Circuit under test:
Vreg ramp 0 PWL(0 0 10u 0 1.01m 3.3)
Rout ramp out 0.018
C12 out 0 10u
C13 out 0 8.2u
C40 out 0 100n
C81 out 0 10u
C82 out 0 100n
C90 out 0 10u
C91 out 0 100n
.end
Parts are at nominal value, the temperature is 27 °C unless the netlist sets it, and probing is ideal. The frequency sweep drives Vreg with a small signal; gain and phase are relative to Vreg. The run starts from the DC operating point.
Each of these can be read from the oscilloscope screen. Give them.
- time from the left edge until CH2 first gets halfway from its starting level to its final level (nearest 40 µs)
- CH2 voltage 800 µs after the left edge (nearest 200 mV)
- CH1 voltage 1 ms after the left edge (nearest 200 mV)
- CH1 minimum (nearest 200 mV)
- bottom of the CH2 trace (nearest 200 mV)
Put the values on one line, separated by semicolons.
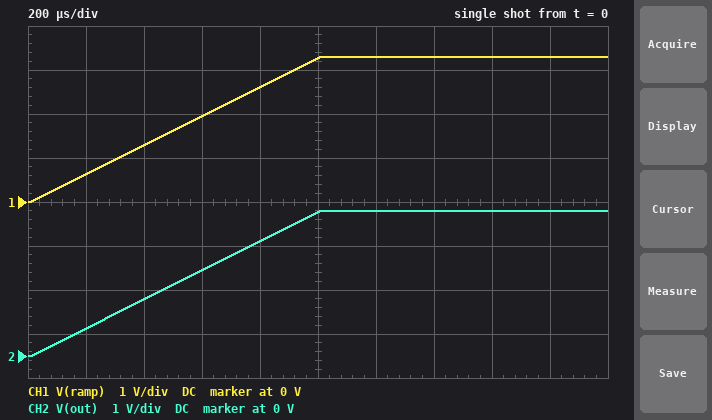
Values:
520 µs; 2.6 V; 3.2 V; 0 V; 0 V
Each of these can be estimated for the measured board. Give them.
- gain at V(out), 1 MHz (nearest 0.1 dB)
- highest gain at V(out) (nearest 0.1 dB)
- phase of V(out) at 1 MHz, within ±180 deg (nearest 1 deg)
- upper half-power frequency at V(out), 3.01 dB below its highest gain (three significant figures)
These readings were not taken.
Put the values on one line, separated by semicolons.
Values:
-13.0 dB; 0 dB; -77 deg; 230 kHz
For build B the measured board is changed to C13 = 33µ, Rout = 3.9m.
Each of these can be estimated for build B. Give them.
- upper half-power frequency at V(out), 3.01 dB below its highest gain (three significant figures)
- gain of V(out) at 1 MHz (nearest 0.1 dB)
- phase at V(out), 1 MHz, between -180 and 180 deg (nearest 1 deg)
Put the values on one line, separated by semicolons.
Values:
645 kHz; -5.3 dB; -57 deg
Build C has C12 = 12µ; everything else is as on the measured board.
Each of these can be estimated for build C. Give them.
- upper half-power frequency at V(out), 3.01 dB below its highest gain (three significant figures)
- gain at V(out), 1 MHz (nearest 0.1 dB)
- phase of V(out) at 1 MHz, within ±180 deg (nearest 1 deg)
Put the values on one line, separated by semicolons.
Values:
218 kHz; -13.4 dB; -78 deg
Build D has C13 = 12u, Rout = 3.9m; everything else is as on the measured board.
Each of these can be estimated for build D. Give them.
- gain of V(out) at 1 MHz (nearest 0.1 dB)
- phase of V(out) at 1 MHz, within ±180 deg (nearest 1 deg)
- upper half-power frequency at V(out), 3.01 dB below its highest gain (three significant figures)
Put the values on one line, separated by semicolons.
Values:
-3.2 dB; -46 deg; 965 kHz
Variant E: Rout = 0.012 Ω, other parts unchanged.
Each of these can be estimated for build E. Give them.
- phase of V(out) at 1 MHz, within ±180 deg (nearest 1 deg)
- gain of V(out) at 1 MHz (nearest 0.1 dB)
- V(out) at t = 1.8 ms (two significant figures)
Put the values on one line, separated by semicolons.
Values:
-71 deg; -9.7 dB; 3.3 V
